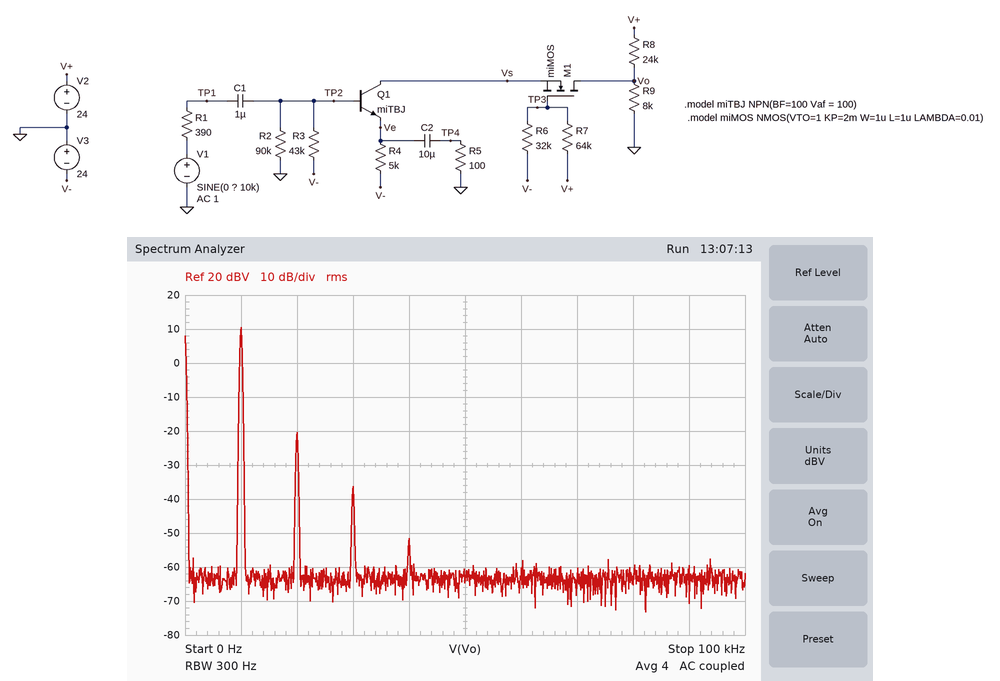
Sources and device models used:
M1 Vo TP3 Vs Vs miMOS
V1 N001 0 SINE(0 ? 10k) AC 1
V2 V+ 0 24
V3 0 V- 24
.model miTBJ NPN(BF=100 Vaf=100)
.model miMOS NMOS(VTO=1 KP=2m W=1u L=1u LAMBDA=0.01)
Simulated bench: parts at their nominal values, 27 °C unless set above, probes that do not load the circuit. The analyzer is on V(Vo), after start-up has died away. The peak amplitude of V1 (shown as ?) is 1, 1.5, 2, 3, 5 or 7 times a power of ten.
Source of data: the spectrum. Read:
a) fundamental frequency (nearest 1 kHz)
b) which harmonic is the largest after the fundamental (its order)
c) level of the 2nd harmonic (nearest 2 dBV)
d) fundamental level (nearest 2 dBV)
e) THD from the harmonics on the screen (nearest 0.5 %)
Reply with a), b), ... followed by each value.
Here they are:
a) 10 kHz
b) 2
c) -20 dBV
d) 10 dBV
e) 3.0 %
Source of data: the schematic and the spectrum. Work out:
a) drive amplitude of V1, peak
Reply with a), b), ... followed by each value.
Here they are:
a) 100 mV
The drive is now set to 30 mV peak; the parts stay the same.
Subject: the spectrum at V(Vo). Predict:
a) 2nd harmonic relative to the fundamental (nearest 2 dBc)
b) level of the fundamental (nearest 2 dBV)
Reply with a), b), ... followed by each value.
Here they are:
a) -42 dBc
b) 0 dBV
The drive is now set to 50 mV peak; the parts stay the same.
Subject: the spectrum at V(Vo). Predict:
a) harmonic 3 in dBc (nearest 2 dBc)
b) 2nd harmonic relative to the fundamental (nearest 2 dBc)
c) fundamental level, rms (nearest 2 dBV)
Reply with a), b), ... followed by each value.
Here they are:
a) -60 dBc
b) -38 dBc
c) 4 dBV
